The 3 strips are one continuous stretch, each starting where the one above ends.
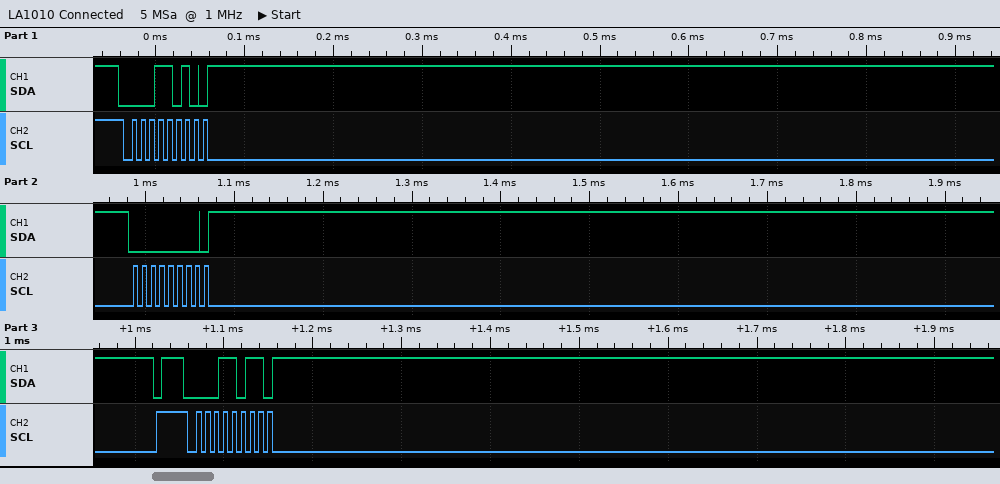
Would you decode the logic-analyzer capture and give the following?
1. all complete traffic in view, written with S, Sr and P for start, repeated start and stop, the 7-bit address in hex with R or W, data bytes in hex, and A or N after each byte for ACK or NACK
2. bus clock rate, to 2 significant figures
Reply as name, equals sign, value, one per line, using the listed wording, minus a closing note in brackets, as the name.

all complete traffic in view, written with S, Sr and P for start, repeated start and stop, the 7-bit address in hex with R or W, data bytes in hex, and A or N after each byte for ACK or NACK = S 0DW A 00 A P S 0DR A
bus clock rate, to 2 significant figures = 100 kHz
